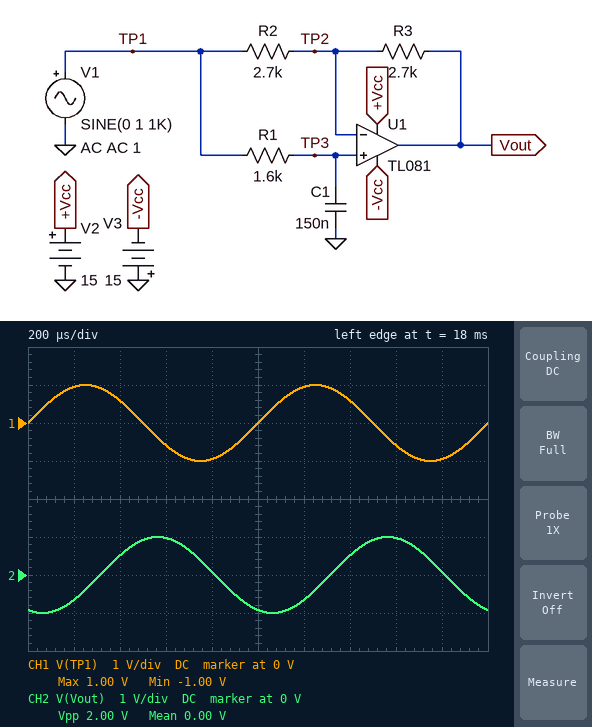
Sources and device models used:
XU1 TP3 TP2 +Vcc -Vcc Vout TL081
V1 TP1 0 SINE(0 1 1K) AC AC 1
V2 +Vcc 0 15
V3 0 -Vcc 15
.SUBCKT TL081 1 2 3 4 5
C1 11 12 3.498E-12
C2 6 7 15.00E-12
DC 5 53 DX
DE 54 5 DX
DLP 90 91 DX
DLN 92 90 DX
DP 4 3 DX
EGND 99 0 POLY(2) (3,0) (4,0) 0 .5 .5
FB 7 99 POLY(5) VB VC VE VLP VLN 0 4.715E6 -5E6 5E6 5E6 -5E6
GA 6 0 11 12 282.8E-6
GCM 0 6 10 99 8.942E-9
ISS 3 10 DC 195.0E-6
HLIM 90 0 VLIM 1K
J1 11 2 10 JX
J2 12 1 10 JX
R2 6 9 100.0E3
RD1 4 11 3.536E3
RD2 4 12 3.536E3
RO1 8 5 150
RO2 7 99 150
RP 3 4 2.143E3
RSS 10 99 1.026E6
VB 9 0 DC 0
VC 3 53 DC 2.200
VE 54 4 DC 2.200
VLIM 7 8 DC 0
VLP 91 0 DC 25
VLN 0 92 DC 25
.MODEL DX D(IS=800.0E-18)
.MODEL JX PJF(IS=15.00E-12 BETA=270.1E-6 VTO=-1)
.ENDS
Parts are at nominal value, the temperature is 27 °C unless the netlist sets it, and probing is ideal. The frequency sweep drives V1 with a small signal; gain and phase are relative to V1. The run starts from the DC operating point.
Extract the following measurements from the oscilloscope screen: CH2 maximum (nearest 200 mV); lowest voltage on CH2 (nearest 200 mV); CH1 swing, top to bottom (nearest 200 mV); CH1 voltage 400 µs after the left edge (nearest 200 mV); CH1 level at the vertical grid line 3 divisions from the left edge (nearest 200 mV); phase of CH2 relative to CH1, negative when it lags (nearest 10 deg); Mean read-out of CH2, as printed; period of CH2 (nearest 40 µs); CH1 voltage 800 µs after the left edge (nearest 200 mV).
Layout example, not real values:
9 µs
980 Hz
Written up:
1.0 V
-1.0 V
2.0 V
600 mV
-600 mV
-110 deg
0.00 V
1.00 ms
-1.0 V
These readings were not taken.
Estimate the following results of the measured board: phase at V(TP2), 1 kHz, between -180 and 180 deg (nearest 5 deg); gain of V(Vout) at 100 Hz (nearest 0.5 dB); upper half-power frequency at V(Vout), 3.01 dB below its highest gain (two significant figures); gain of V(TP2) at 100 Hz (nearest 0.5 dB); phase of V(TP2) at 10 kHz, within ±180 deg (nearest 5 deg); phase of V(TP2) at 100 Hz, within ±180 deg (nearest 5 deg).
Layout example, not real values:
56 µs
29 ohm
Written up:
-55 deg
0 dB
2.2 MHz
0 dB
-85 deg
-10 deg
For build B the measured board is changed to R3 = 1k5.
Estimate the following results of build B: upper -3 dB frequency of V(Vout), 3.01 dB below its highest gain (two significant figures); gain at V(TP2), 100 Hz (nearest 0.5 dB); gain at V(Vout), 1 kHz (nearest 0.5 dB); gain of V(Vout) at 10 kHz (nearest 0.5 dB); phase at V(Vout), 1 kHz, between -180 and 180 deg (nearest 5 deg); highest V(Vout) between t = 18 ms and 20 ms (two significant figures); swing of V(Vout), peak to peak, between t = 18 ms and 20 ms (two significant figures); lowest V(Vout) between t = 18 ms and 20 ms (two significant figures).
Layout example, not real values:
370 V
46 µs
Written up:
1.1 kHz
0 dB
-3.0 dB
-5.0 dB
-95 deg
720 mV
1.4 V
-720 mV
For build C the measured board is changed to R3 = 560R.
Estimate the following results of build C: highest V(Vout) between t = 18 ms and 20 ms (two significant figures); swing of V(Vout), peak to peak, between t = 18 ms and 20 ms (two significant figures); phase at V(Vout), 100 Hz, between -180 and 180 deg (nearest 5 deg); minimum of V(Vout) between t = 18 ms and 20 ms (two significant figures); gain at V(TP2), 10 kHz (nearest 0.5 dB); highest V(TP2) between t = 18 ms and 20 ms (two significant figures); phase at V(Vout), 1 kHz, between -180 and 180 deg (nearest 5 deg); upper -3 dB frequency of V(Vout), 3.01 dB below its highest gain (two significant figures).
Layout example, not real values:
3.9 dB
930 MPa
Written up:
580 mV
1.2 V
-10 deg
-580 mV
-23.5 dB
550 mV
-75 deg
690 Hz
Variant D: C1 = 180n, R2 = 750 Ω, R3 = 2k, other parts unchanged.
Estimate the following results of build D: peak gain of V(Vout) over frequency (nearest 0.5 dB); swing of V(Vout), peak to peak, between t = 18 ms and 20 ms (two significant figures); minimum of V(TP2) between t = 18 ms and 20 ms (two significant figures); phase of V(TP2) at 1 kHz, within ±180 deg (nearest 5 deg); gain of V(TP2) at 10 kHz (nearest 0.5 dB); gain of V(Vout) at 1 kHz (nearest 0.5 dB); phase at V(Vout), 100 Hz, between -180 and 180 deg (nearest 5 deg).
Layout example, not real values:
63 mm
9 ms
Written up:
8.5 dB
4.8 V
-480 mV
-60 deg
-26.5 dB
7.5 dB
-35 deg
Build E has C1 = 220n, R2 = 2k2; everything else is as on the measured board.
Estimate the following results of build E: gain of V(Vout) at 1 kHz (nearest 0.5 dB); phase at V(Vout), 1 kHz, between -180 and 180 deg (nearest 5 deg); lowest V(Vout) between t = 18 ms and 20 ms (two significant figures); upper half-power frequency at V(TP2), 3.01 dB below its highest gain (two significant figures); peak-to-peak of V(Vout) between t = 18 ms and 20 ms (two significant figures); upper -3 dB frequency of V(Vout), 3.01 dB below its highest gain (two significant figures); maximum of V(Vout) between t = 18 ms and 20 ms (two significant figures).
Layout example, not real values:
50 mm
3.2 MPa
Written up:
1.5 dB
-135 deg
-1.2 V
450 Hz
2.4 V
1.9 MHz
1.2 V
